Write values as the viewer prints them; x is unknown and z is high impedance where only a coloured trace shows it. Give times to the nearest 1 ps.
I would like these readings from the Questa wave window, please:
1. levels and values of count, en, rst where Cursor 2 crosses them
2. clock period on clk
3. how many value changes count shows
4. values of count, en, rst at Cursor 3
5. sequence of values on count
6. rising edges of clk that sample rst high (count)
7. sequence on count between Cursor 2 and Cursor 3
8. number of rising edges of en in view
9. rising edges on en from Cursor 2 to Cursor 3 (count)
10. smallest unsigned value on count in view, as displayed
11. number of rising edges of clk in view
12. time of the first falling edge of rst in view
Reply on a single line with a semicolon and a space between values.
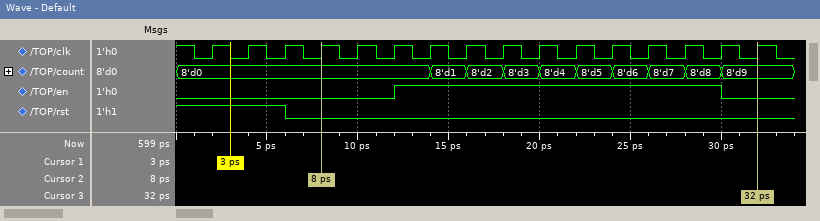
count=8'd0, en=0, rst=0; 2 ps; 9; count=8'd9, en=0, rst=0; 8'd0, 8'd1, 8'd2, 8'd3, 8'd4, 8'd5, 8'd6, 8'd7, 8'd8, 8'd9; 3; 8'd0, 8'd1, 8'd2, 8'd3, 8'd4, 8'd5, 8'd6, 8'd7, 8'd8, 8'd9; 1; 1; 8'd0; 16; 6 ps
